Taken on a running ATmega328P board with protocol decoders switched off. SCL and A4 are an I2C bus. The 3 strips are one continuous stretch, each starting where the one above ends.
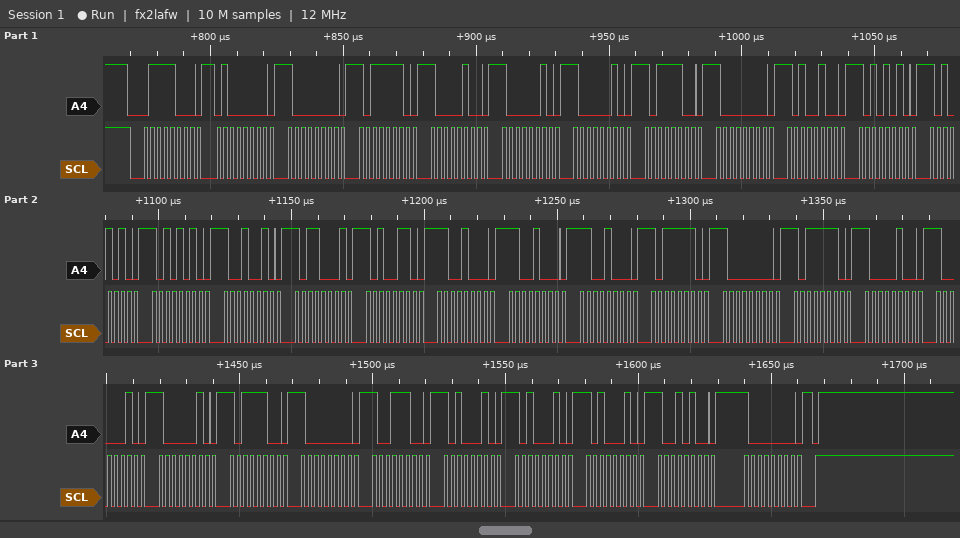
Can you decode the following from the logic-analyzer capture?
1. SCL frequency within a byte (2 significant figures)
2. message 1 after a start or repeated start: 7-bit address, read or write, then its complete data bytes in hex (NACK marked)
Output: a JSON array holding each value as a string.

["400 kHz", "0x3C write: 40 80 BE 84 82 82 BC 80 A4 AA AA AA 92 B1 A6 C8 C8 C8 BE 80 BE 84 82 82 BC 80 9C A2 A2 A2 94 80"]
